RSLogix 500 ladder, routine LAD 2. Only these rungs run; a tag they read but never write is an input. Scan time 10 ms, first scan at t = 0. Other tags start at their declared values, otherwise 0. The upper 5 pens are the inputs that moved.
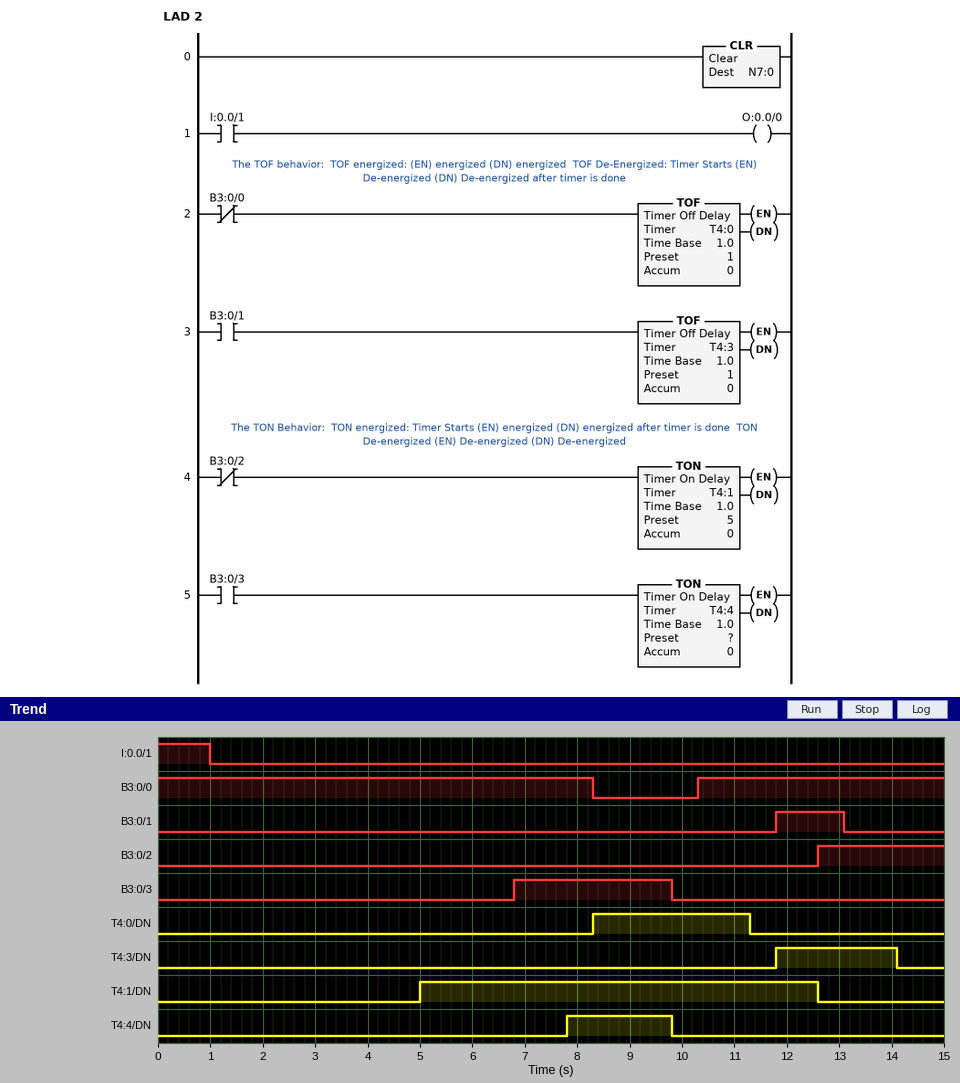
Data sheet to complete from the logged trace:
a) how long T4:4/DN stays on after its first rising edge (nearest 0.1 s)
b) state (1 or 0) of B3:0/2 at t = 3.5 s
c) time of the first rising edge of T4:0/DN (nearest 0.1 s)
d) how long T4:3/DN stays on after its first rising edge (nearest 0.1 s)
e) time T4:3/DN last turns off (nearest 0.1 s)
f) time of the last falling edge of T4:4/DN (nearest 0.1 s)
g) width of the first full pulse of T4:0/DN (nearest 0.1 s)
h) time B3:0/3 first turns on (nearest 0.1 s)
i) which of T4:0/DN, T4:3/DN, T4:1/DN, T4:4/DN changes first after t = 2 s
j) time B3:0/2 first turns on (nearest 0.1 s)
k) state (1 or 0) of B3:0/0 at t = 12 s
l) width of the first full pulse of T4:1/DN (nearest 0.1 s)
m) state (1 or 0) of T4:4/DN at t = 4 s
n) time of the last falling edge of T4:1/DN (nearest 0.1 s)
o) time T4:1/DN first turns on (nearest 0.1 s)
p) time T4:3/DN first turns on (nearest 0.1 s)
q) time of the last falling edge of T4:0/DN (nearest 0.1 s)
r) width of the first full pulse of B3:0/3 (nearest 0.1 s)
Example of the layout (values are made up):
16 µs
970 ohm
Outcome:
2.0 s
0
8.3 s
2.3 s
14.1 s
9.8 s
3.0 s
6.8 s
T4:1/DN
12.6 s
1
7.6 s
0
12.6 s
5.0 s
11.8 s
11.3 s
3.0 s
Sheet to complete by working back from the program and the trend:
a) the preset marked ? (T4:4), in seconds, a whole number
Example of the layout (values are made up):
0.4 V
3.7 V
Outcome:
1 s
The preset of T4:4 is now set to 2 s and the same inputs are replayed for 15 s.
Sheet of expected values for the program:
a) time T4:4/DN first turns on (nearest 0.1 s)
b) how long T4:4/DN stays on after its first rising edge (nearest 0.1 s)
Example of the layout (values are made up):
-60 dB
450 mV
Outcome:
8.8 s
1.0 s
